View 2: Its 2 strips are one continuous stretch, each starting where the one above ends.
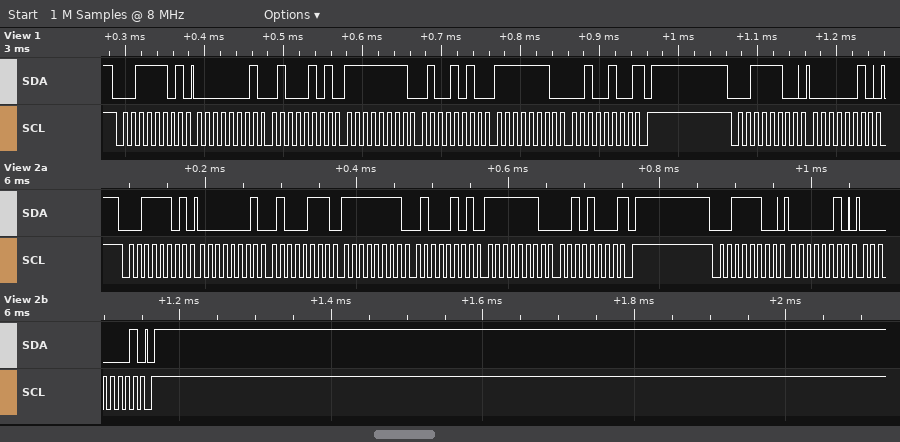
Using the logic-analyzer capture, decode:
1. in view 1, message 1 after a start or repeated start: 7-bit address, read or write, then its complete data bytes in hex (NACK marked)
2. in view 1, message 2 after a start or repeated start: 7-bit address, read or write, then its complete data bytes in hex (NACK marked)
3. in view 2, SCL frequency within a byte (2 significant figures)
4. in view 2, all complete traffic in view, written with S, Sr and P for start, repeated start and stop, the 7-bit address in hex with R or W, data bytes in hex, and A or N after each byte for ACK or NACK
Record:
0x1E read: 01 45 FF 4A FE 24 NACK
0x1E write: 02
100 kHz
S 1ER A 01 A 47 A FF A 45 A FE A 28 N P S 1EW A 02 A 01 A P
